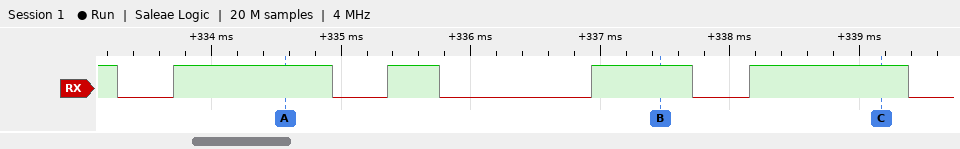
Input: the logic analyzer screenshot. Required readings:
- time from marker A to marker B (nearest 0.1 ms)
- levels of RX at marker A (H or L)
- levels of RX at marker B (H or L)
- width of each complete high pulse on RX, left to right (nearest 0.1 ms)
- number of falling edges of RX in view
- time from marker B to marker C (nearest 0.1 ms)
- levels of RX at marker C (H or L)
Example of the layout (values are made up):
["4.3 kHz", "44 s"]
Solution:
["2.9 ms", "RX=H", "RX=H", "1.2 ms, 0.4 ms, 0.8 ms, 1.2 ms", "5", "1.7 ms", "RX=H"]
